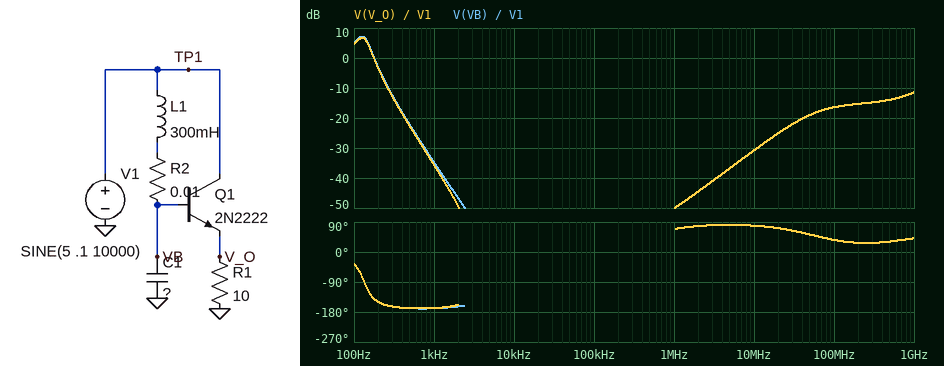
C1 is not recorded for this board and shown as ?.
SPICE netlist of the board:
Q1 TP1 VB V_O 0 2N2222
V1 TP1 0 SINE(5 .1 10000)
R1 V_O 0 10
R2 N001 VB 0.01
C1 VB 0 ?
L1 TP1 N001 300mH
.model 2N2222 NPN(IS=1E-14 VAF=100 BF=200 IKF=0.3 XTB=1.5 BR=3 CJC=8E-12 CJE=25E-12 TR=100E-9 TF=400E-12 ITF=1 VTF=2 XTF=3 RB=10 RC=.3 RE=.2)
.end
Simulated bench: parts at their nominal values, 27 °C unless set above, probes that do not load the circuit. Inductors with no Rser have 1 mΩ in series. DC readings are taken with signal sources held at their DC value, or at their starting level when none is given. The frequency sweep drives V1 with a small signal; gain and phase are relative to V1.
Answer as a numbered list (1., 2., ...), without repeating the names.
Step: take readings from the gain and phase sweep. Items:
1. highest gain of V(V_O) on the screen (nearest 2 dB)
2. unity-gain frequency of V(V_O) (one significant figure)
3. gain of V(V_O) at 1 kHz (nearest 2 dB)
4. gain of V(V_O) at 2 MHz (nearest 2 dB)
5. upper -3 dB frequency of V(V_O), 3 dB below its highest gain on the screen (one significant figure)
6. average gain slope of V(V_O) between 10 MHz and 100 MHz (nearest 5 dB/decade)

1. 6 dB
2. 200 Hz
3. -36 dB
4. -44 dB
5. 200 Hz
6. 15 dB/decade
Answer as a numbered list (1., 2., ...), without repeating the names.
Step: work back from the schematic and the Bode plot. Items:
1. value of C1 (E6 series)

1. 4.7 µF
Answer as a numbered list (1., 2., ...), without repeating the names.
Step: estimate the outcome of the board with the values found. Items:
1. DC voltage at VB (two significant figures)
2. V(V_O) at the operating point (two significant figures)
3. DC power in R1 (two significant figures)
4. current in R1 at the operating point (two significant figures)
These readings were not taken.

1. 5.0 V
2. 4.0 V
3. 1.6 W
4. 400 mA
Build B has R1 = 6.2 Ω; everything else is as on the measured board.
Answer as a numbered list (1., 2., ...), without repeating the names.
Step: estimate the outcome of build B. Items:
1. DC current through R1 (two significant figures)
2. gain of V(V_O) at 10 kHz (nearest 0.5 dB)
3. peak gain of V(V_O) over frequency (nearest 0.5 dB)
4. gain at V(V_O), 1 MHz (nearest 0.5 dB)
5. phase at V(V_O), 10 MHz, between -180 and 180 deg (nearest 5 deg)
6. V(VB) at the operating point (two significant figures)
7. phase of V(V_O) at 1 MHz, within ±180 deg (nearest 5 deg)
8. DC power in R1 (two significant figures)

1. 630 mA
2. -55.0 dB
3. 0.5 dB
4. -42.5 dB
5. 70 deg
6. 5.0 V
7. 75 deg
8. 2.5 W
